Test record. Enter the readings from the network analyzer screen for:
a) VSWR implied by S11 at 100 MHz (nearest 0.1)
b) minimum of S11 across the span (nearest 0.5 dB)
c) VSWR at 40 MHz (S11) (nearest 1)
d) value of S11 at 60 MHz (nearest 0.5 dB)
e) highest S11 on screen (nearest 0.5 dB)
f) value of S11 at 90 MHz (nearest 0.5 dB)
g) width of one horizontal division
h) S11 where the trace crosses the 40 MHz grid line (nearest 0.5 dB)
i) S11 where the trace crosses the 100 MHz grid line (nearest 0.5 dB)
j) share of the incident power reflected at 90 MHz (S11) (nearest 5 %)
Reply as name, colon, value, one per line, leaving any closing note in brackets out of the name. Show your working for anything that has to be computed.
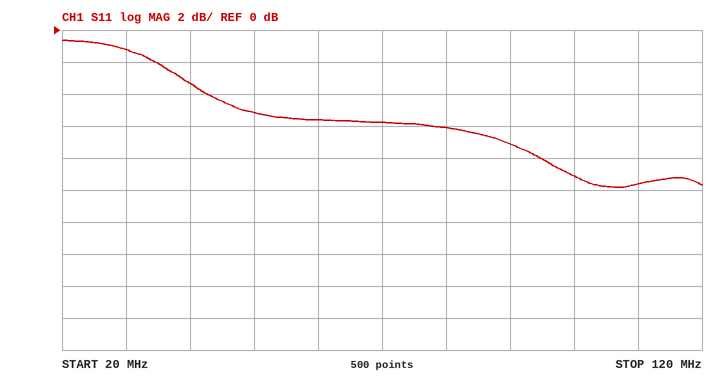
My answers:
VSWR implied by S11 at 100 MHz: |Γ| = 10^(-9/20) = 0.3548; VSWR = (1 + 0.3548)/(1 − 0.3548) ≈ 2.1
minimum of S11 across the span: -10.0 dB
VSWR at 40 MHz (S11): |Γ| = 10^(-3.5/20) = 0.6683; VSWR = (1 + 0.6683)/(1 − 0.6683) ≈ 5
value of S11 at 60 MHz: -5.5 dB
highest S11 on screen: -0.5 dB
value of S11 at 90 MHz: -7.0 dB
width of one horizontal division: 10 MHz
S11 where the trace crosses the 40 MHz grid line: -3.5 dB
S11 where the trace crosses the 100 MHz grid line: -9.0 dB
share of the incident power reflected at 90 MHz (S11): 10^(-7/10) ≈ 20 %
